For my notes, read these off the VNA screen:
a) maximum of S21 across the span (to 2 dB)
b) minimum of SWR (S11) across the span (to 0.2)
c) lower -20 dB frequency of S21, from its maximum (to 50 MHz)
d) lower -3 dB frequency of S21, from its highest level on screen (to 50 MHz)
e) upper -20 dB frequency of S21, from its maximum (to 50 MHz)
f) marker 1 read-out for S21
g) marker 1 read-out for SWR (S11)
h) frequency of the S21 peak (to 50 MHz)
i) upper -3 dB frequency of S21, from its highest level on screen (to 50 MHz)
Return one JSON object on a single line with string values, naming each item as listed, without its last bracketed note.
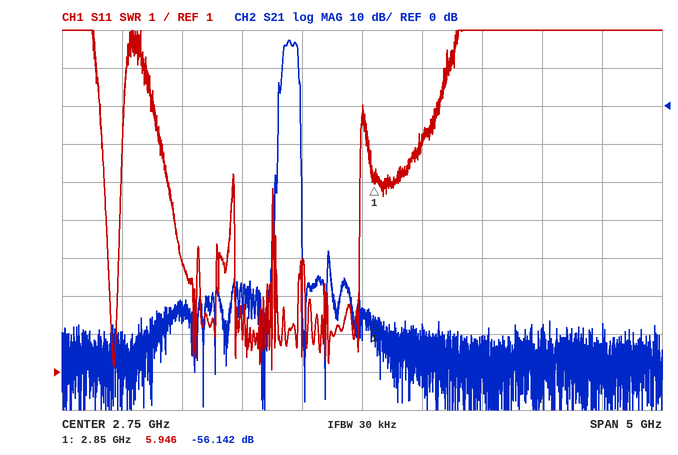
{"maximum of S21 across the span": "18 dB", "minimum of SWR (S11) across the span": "1.0", "lower -20 dB frequency of S21, from its maximum": "2.05 GHz", "lower -3 dB frequency of S21, from its highest level on screen": "2.10 GHz", "upper -20 dB frequency of S21, from its maximum": "2.25 GHz", "marker 1 read-out for S21": "-56.142 dB", "marker 1 read-out for SWR": "5.946", "frequency of the S21 peak": "2.15 GHz", "upper -3 dB frequency of S21, from its highest level on screen": "2.20 GHz"}
